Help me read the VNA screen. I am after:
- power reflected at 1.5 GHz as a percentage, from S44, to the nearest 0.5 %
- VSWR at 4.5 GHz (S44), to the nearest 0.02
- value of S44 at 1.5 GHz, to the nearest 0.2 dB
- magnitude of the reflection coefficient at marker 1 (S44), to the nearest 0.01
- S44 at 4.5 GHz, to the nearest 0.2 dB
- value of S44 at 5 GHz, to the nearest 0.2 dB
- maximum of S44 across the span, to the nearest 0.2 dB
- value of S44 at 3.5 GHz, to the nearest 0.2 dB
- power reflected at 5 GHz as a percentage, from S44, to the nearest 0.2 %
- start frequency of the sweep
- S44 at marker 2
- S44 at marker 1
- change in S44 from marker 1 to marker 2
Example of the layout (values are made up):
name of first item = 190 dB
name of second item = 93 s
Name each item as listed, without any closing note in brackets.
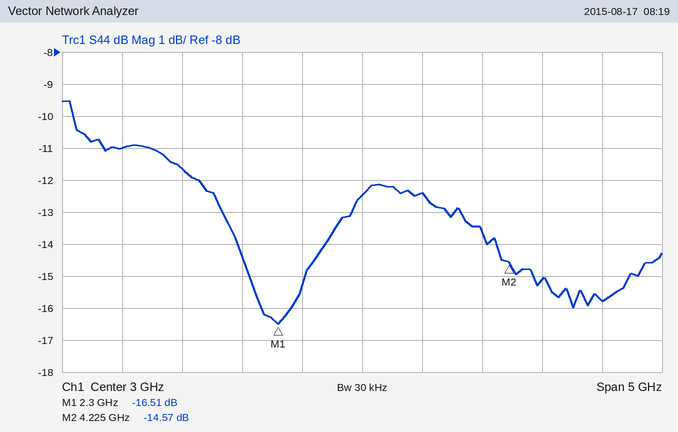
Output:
power reflected at 1.5 GHz as a percentage, from S44, to the nearest 0.5 % = 7.0 %
VSWR at 4.5 GHz (S44), to the nearest 0.02 = 1.42
value of S44 at 1.5 GHz, to the nearest 0.2 dB = -11.6 dB
magnitude of the reflection coefficient at marker 1 (S44), to the nearest 0.01 = 0.15
S44 at 4.5 GHz, to the nearest 0.2 dB = -15.2 dB
value of S44 at 5 GHz, to the nearest 0.2 dB = -15.8 dB
maximum of S44 across the span, to the nearest 0.2 dB = -9.6 dB
value of S44 at 3.5 GHz, to the nearest 0.2 dB = -12.4 dB
power reflected at 5 GHz as a percentage, from S44, to the nearest 0.2 % = 2.6 %
start frequency of the sweep = 500 MHz
S44 at marker 2 = -14.57 dB
S44 at marker 1 = -16.51 dB
change in S44 from marker 1 to marker 2 = 1.94 dB
